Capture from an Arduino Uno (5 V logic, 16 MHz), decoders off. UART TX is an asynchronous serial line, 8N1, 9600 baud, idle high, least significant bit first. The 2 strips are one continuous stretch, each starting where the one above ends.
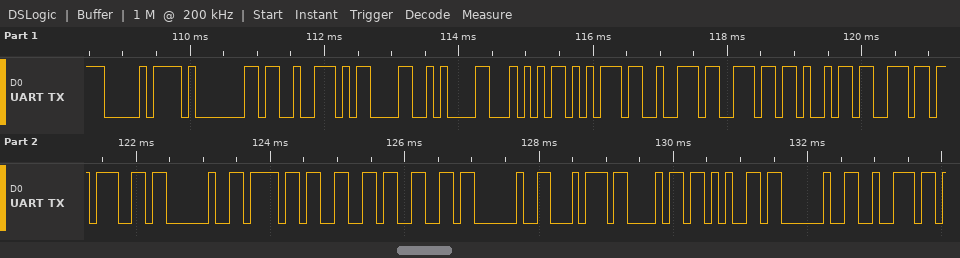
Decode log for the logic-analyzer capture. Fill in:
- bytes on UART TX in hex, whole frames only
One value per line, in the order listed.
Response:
0xD0 0x01 0x93 0x0D 0x0A 0x54 0x75 0x72 0x6E 0x69 0x6E 0x67 0x20 0x6F 0x66 0x66 0x20 0x74 0x68 0x65 0x20 0x72
